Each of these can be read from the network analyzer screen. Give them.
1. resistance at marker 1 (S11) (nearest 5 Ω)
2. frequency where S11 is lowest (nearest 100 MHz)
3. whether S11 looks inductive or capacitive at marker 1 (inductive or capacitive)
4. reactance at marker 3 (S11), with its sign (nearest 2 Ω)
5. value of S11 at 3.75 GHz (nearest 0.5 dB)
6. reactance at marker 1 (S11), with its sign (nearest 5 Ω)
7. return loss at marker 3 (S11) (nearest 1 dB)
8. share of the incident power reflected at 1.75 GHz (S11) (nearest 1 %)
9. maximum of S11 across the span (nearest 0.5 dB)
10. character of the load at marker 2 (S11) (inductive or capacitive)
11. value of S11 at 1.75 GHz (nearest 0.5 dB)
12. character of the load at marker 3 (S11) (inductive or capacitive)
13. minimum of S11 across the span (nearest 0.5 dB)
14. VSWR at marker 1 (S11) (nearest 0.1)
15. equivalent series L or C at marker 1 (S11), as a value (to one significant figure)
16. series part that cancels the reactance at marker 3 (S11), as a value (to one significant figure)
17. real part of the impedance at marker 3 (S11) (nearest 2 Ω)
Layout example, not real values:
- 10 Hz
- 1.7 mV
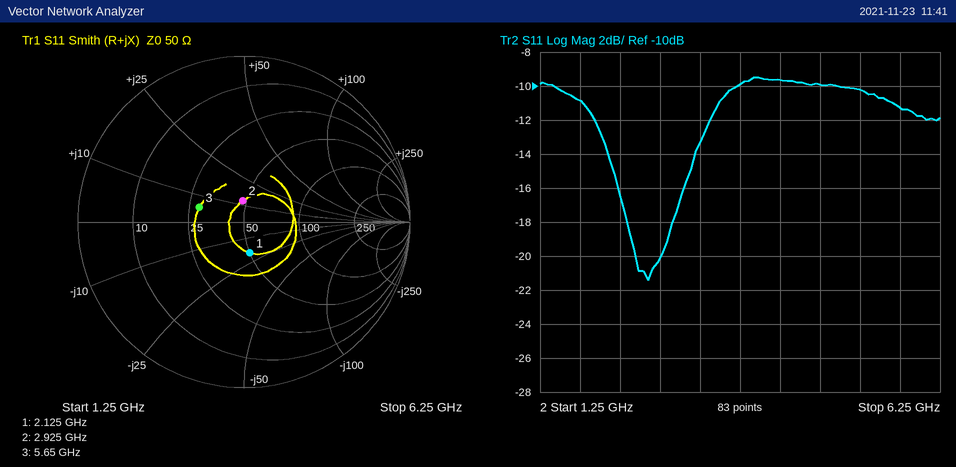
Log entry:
- 50 Ω
- 2.6 GHz
- capacitive
- +6 Ω
- -10.0 dB
- -20 Ω
- 11 dB
- 8 %
- -9.5 dB
- inductive
- -11.0 dB
- inductive
- -21.5 dB
- 1.5
- 4 pF
- 5 pF
- 28 Ω
